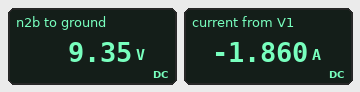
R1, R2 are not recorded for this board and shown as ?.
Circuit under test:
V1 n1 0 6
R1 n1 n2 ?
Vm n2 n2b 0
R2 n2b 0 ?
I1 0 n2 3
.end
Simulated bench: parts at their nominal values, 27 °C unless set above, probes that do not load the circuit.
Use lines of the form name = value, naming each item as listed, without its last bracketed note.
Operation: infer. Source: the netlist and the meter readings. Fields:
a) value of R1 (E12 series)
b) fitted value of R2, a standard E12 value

value of R1 = 1.8 Ω
fitted value of R2, a standard E12 value = 8.2 Ω
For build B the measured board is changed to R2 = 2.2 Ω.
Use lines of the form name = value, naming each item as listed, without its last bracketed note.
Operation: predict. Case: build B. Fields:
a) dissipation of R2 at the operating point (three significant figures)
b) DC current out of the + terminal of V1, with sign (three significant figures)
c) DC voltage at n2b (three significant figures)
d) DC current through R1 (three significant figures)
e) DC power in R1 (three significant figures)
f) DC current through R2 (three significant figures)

dissipation of R2 at the operating point = 17.9 W
DC current out of the + terminal of V1, with sign = -150 mA
DC voltage at n2b = 6.27 V
DC current through R1 = 150 mA
DC power in R1 = 40.5 mW
DC current through R2 = 2.85 A
